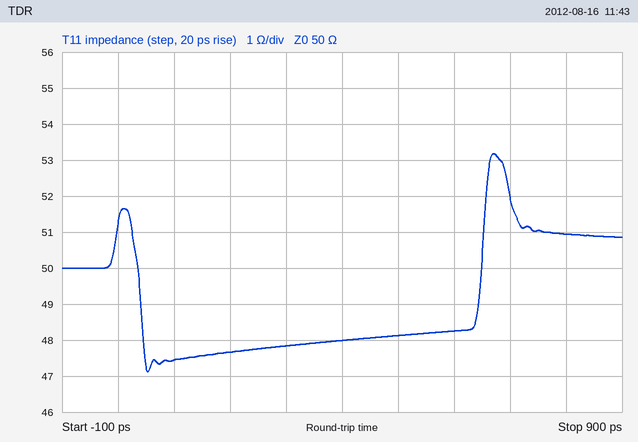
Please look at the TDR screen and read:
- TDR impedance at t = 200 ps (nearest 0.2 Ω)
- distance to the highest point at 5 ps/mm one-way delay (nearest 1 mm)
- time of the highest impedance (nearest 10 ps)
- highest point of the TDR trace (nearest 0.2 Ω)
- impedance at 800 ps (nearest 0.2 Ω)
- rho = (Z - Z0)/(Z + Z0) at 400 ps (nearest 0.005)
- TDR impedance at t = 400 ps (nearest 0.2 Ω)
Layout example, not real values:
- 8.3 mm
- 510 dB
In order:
- 47.6 Ω
- 67 mm
- 670 ps
- 53.2 Ω
- 51.0 Ω
- -0.020
- 48.0 Ω
